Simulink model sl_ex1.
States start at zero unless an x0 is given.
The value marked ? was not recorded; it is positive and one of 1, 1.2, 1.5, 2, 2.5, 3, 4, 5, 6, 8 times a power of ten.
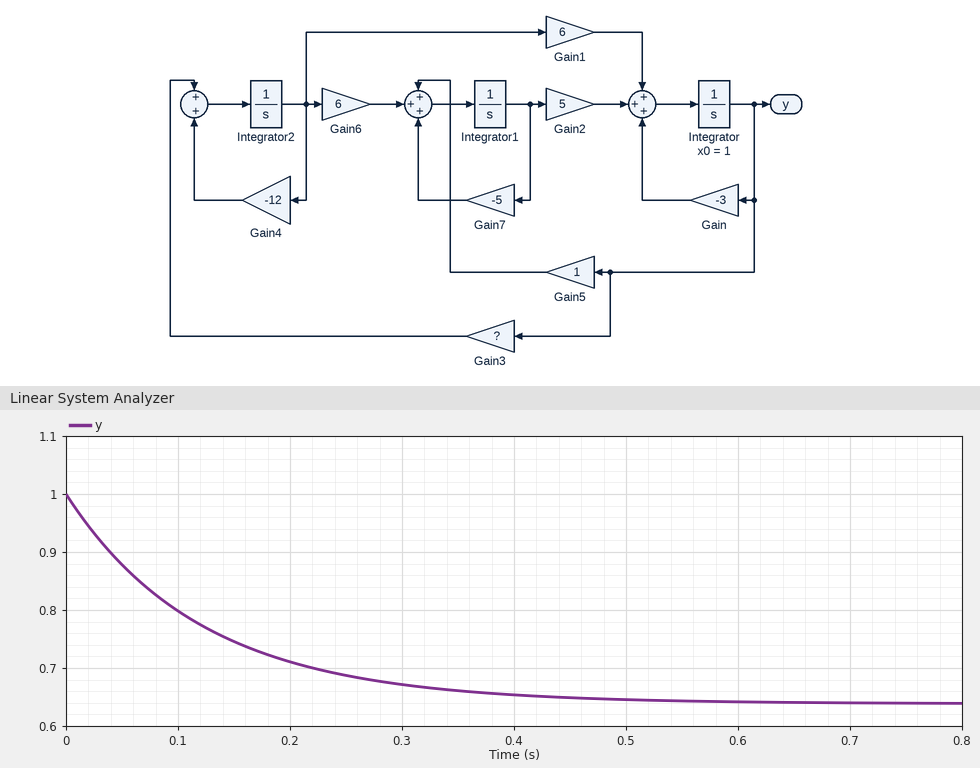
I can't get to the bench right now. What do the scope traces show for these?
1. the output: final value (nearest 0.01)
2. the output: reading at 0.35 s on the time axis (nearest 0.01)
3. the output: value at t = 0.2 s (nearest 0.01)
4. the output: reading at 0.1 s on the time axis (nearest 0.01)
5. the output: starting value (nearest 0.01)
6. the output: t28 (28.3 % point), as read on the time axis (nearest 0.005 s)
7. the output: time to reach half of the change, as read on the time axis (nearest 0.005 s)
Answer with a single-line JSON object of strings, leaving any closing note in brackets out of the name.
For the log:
{"the output: final value": "0.64", "the output: reading at 0.35 s on the time axis": "0.66", "the output: value at t = 0.2 s": "0.71", "the output: reading at 0.1 s on the time axis": "0.80", "the output: starting value": "1.00", "the output: t28 (28.3 % point), as read on the time axis": "0.040 s", "the output: time to reach half of the change, as read on the time axis": "0.085 s"}
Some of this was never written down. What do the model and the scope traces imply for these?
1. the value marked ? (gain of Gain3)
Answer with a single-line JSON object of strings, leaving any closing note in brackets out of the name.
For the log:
{"the value marked ?": "2"}
